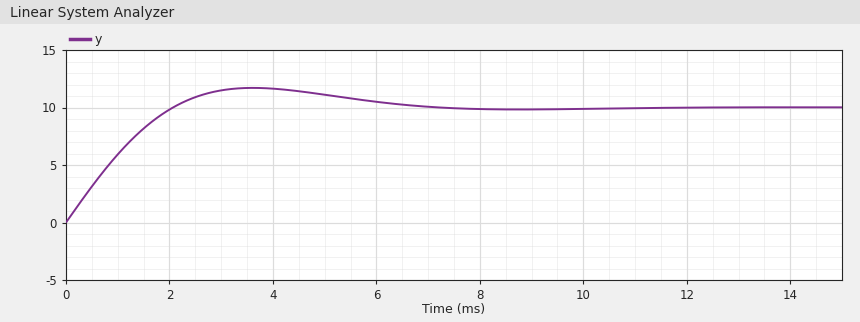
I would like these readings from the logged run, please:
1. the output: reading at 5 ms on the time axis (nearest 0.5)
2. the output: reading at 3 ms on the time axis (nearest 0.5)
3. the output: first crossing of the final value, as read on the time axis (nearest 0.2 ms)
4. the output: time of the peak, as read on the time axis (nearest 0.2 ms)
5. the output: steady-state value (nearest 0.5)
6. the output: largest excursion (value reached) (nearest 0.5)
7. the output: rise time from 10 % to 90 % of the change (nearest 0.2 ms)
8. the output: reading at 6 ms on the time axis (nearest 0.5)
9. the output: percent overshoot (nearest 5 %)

11.0
11.5
2.0 ms
3.6 ms
10.0
11.5
1.6 ms
10.5
15 %
